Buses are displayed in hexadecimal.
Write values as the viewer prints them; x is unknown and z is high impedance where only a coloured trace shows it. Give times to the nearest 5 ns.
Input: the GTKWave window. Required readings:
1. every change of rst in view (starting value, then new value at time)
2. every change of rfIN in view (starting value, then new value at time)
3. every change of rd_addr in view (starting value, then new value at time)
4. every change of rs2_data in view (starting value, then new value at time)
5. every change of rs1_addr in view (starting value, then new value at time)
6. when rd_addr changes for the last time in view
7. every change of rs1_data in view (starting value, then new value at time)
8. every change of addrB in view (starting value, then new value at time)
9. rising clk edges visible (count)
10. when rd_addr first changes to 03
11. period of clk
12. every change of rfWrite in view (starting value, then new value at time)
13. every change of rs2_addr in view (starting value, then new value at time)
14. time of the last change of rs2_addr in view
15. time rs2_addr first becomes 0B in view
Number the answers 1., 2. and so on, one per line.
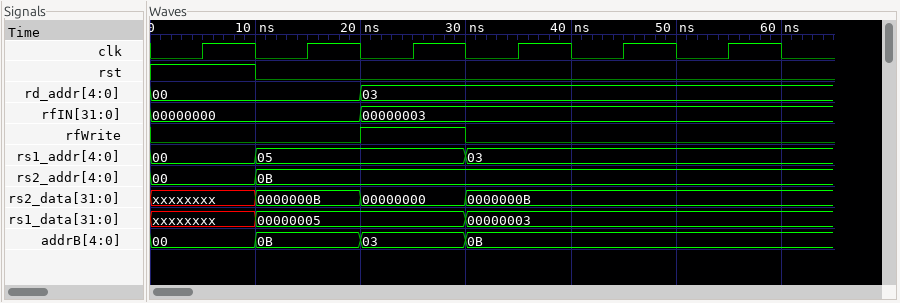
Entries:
1. 1, 0 at 10 ns
2. 00000000, 00000003 at 20 ns
3. 00, 03 at 20 ns
4. xxxxxxxx, 0000000B at 10 ns, 00000000 at 20 ns, 0000000B at 30 ns
5. 00, 05 at 10 ns, 03 at 30 ns
6. 20 ns
7. xxxxxxxx, 00000005 at 10 ns, 00000003 at 30 ns
8. 00, 0B at 10 ns, 03 at 20 ns, 0B at 30 ns
9. 6
10. 20 ns
11. 10 ns
12. 0, 1 at 20 ns, 0 at 30 ns
13. 00, 0B at 10 ns
14. 10 ns
15. 10 ns
